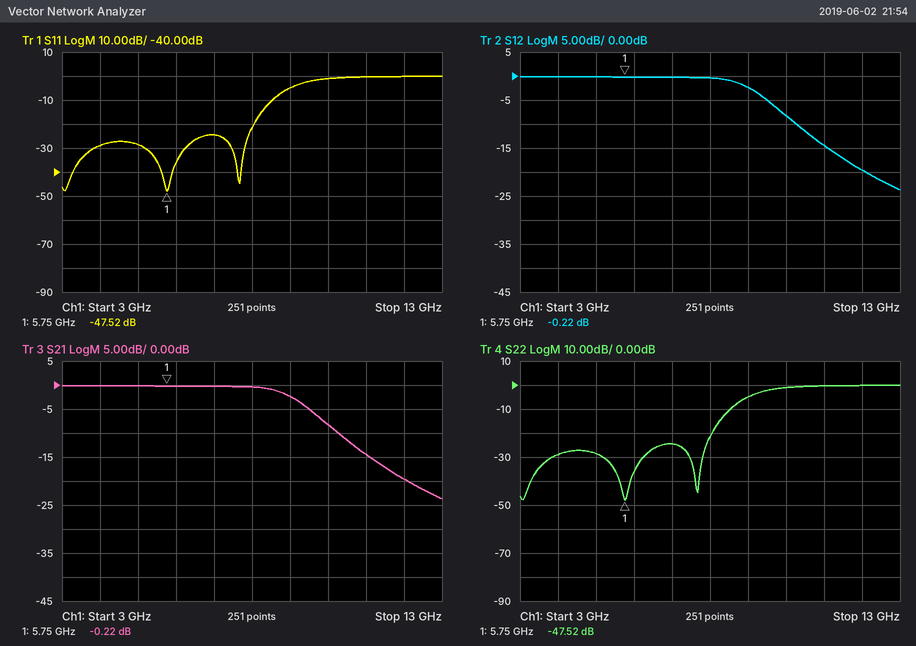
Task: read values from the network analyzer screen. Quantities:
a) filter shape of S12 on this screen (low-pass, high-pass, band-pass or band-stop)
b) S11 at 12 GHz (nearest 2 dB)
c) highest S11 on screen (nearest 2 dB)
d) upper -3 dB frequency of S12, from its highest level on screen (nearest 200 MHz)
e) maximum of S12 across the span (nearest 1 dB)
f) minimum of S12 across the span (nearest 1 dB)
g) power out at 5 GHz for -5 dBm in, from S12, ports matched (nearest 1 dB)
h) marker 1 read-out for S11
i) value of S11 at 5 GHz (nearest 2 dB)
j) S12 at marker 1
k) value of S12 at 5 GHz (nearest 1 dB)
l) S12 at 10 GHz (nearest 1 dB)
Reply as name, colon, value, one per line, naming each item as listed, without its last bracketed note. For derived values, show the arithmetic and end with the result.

filter shape of S12 on this screen: low-pass
S11 at 12 GHz: 0 dB
highest S11 on screen: 0 dB
upper -3 dB frequency of S12, from its highest level on screen: 9.2 GHz
maximum of S12 across the span: 0 dB
minimum of S12 across the span: -24 dB
power out at 5 GHz for -5 dBm in, from S12, ports matched: -5 dBm + (0 dB) = -5 dBm
marker 1 read-out for S11: -47.52 dB
value of S11 at 5 GHz: -28 dB
S12 at marker 1: -0.22 dB
value of S12 at 5 GHz: 0 dB
S12 at 10 GHz: -8 dB
